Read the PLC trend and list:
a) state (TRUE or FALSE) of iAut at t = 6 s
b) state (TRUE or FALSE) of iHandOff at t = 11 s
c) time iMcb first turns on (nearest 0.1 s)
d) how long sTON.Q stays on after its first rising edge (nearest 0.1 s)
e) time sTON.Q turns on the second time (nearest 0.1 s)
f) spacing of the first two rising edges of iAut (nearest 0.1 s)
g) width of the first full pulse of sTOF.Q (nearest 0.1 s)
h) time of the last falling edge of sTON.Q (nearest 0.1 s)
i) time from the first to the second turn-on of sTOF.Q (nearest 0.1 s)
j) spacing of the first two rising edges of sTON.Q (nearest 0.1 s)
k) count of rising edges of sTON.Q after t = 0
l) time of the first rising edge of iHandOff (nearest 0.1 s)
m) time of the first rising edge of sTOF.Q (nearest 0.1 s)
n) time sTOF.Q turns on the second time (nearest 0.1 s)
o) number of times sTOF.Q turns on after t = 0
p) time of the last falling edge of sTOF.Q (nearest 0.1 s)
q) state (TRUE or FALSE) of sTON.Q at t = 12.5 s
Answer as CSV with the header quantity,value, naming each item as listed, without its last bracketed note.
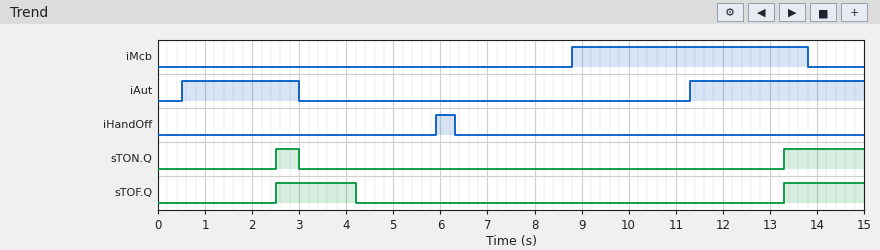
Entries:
quantity,value
state (TRUE or FALSE) of iAut at t = 6 s,FALSE
state (TRUE or FALSE) of iHandOff at t = 11 s,FALSE
time iMcb first turns on,8.8 s
how long sTON.Q stays on after its first rising edge,0.5 s
time sTON.Q turns on the second time,13.3 s
spacing of the first two rising edges of iAut,10.8 s
width of the first full pulse of sTOF.Q,1.7 s
time of the last falling edge of sTON.Q,3.0 s
time from the first to the second turn-on of sTOF.Q,10.8 s
spacing of the first two rising edges of sTON.Q,10.8 s
count of rising edges of sTON.Q after t = 0,2
time of the first rising edge of iHandOff,5.9 s
time of the first rising edge of sTOF.Q,2.5 s
time sTOF.Q turns on the second time,13.3 s
number of times sTOF.Q turns on after t = 0,2
time of the last falling edge of sTOF.Q,4.2 s
state (TRUE or FALSE) of sTON.Q at t = 12.5 s,FALSE
